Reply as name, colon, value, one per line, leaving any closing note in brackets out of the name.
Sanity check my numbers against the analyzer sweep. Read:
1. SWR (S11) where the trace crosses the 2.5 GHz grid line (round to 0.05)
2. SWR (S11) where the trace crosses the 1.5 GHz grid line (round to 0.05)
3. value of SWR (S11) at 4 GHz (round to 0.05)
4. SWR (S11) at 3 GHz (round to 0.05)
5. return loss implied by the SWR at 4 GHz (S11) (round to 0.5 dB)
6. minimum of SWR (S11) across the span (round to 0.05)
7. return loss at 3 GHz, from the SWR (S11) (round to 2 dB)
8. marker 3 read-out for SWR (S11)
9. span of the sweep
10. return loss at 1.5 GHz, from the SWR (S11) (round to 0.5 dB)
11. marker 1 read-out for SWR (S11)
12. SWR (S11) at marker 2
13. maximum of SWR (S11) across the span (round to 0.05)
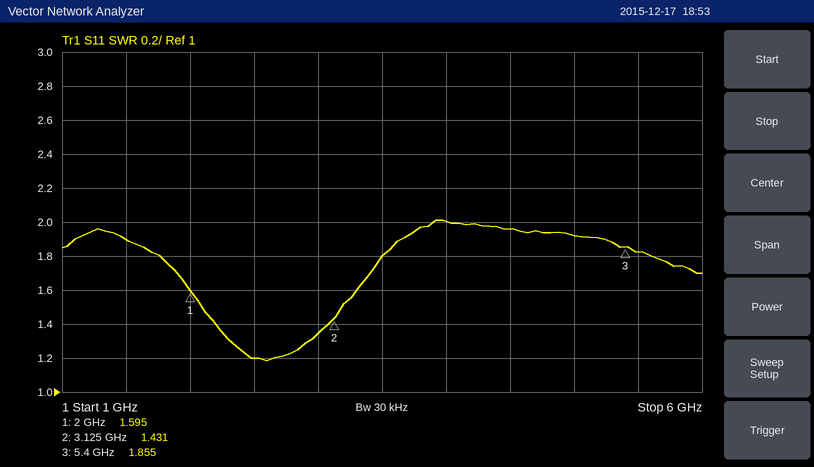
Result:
SWR (S11) where the trace crosses the 2.5 GHz grid line: 1.20
SWR (S11) where the trace crosses the 1.5 GHz grid line: 1.90
value of SWR (S11) at 4 GHz: 2.00
SWR (S11) at 3 GHz: 1.35
return loss implied by the SWR at 4 GHz (S11): 9.5 dB
minimum of SWR (S11) across the span: 1.20
return loss at 3 GHz, from the SWR (S11): 16 dB
marker 3 read-out for SWR: 1.855
span of the sweep: 5 GHz
return loss at 1.5 GHz, from the SWR (S11): 10.0 dB
marker 1 read-out for SWR: 1.595
SWR (S11) at marker 2: 1.431
maximum of SWR (S11) across the span: 2.00
